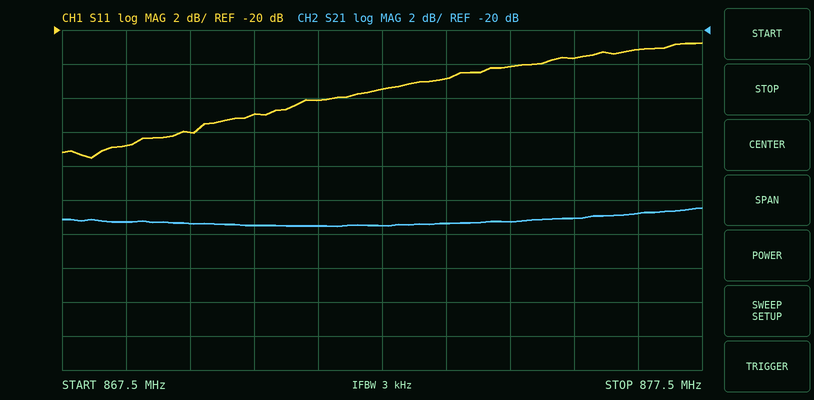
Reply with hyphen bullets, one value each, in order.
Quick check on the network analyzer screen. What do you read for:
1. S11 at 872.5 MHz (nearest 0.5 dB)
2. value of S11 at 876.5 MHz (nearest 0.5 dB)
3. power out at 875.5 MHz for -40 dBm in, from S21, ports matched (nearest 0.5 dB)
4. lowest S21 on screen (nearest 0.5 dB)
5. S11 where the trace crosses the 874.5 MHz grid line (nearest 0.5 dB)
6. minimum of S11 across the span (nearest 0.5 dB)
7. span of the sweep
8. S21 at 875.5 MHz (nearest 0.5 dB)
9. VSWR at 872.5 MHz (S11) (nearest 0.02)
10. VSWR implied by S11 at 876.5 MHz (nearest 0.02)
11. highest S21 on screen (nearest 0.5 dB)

- -23.5 dB
- -21.0 dB
- -71.0 dBm
- -31.5 dB
- -22.0 dB
- -27.5 dB
- 10 MHz
- -31.0 dB
- 1.14
- 1.20
- -30.5 dB
